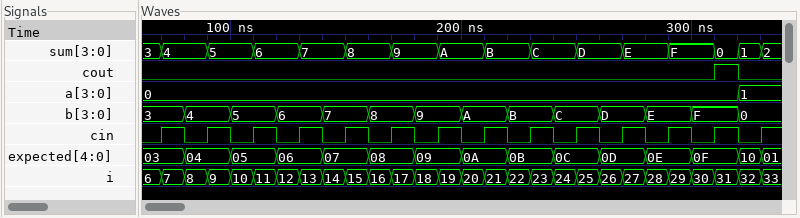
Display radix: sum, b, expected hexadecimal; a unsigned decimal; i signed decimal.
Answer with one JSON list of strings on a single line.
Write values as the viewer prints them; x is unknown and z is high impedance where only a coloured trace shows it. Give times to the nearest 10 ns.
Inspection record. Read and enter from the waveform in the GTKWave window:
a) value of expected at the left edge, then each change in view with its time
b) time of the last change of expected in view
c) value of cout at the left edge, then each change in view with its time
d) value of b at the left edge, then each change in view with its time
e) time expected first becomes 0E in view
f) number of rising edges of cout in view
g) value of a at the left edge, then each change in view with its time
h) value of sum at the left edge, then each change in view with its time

["03, 04 at 80 ns, 05 at 100 ns, 06 at 120 ns, 07 at 140 ns, 08 at 160 ns, 09 at 180 ns, 0A at 200 ns, 0B at 220 ns, 0C at 240 ns, 0D at 260 ns, 0E at 280 ns, 0F at 300 ns, 10 at 320 ns, 01 at 330 ns", "330 ns", "0, 1 at 310 ns, 0 at 320 ns", "3, 4 at 80 ns, 5 at 100 ns, 6 at 120 ns, 7 at 140 ns, 8 at 160 ns, 9 at 180 ns, A at 200 ns, B at 220 ns, C at 240 ns, D at 260 ns, E at 280 ns, F at 300 ns, 0 at 320 ns", "280 ns", "1", "0, 1 at 320 ns", "3, 4 at 70 ns, 5 at 90 ns, 6 at 110 ns, 7 at 130 ns, 8 at 150 ns, 9 at 170 ns, A at 190 ns, B at 210 ns, C at 230 ns, D at 250 ns, E at 270 ns, F at 290 ns, 0 at 310 ns, 1 at 320 ns, 2 at 330 ns"]
